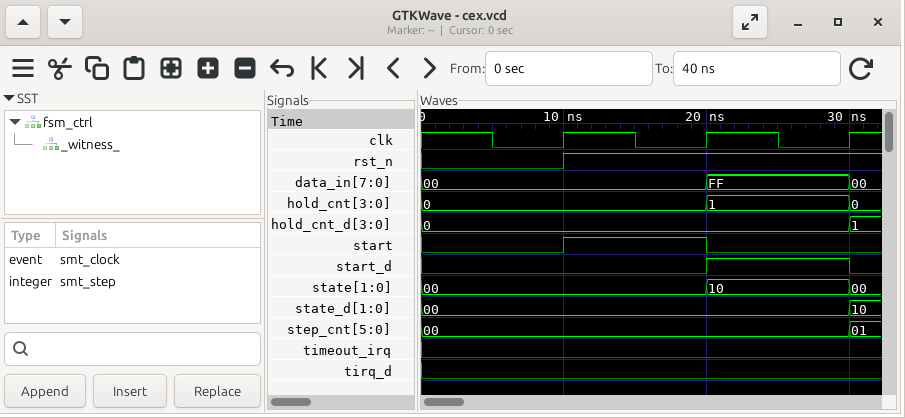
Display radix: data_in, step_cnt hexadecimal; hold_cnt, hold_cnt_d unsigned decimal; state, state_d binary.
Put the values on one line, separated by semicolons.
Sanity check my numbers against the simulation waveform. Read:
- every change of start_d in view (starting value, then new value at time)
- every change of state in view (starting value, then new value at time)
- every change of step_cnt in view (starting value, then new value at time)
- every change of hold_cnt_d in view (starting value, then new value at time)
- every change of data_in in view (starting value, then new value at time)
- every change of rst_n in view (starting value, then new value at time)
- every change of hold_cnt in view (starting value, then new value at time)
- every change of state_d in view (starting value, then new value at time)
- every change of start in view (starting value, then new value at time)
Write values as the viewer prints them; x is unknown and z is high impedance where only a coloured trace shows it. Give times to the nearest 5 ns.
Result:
0, 1 at 20 ns, 0 at 30 ns; 00, 10 at 20 ns, 00 at 30 ns; 00, 01 at 30 ns; 0, 1 at 30 ns; 00, FF at 20 ns, 00 at 30 ns; 0, 1 at 10 ns; 0, 1 at 20 ns, 0 at 30 ns; 00, 10 at 30 ns; 0, 1 at 10 ns, 0 at 20 ns
